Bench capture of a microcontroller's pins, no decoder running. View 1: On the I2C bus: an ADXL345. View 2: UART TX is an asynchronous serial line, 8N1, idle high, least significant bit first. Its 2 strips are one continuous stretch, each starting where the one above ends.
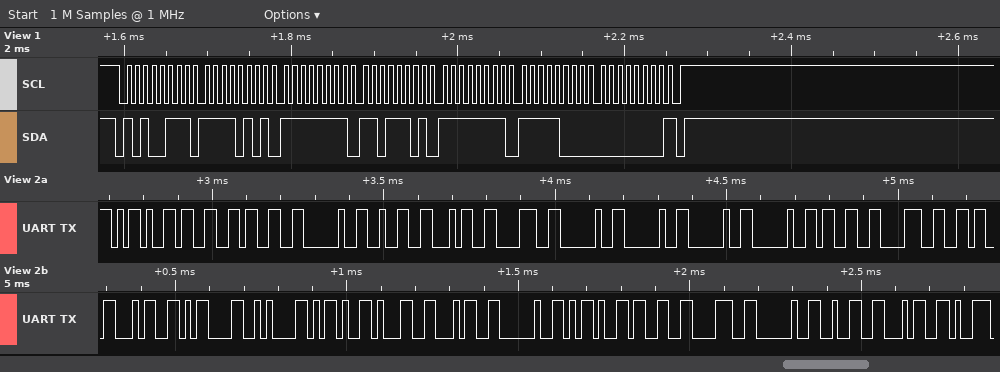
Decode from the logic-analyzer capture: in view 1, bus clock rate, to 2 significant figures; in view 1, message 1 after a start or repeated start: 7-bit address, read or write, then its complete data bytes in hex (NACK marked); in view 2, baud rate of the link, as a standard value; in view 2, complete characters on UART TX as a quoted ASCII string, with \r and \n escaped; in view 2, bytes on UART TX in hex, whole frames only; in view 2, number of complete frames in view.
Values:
100 kHz
0x53 read: F5 FF DD FF F8 00 NACK
57600 baud
"-33 248    3864\r\n-14 -38 24"
0x2D 0x33 0x33 0x20 0x32 0x34 0x38 0x20 0x20 0x20 0x20 0x33 0x38 0x36 0x34 0x0D 0x0A 0x2D 0x31 0x34 0x20 0x2D 0x33 0x38 0x20 0x32 0x34
27
